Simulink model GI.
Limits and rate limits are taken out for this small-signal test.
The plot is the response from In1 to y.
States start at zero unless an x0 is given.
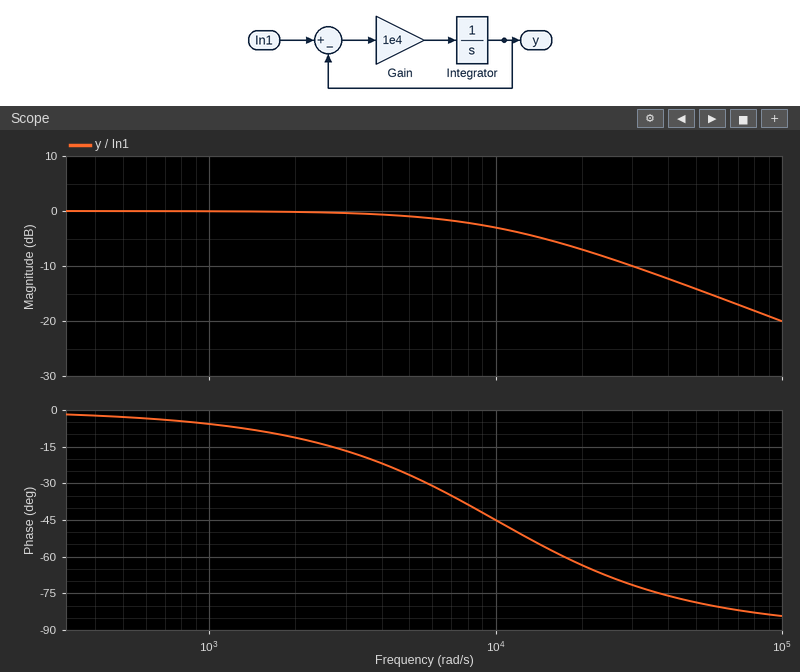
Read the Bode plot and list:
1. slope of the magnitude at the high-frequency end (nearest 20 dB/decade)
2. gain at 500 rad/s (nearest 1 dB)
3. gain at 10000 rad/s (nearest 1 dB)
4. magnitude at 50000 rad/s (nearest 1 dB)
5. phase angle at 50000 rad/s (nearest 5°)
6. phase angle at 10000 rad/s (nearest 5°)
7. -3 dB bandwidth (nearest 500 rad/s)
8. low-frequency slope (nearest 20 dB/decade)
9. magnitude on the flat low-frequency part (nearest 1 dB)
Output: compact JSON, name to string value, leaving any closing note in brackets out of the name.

{"slope of the magnitude at the high-frequency end": "-20 dB/decade", "gain at 500 rad/s": "0 dB", "gain at 10000 rad/s": "-3 dB", "magnitude at 50000 rad/s": "-14 dB", "phase angle at 50000 rad/s": "-80°", "phase angle at 10000 rad/s": "-45°", "-3 dB bandwidth": "10000 rad/s", "low-frequency slope": "0 dB/decade", "magnitude on the flat low-frequency part": "0 dB"}
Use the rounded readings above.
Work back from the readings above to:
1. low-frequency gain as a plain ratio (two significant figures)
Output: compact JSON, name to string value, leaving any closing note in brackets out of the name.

{"low-frequency gain as a plain ratio": "1.0"}
